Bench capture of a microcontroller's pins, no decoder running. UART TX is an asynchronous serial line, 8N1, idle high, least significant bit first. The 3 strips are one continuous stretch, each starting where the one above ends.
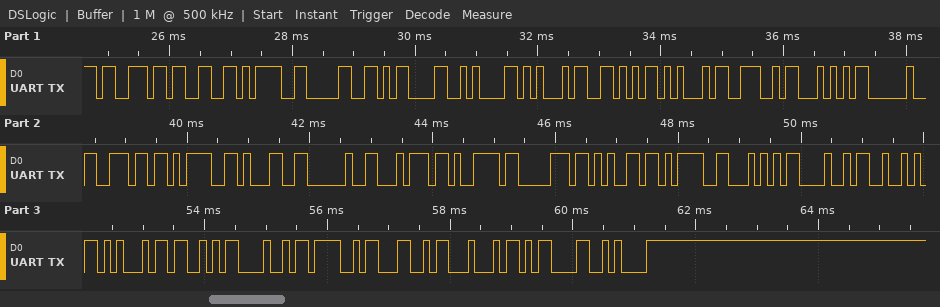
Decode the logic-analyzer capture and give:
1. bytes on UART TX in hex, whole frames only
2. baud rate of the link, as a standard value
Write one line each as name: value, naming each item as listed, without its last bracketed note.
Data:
bytes on UART TX in hex, whole frames only: 73 33 3D 30 0D 0A 45 56 45 4E 54 20 6E 3D 31 20 74 79 70 65 3D 54 48 52 45 53 48 4F 4C 44 0D 0A
baud rate of the link, as a standard value: 9600 baud
